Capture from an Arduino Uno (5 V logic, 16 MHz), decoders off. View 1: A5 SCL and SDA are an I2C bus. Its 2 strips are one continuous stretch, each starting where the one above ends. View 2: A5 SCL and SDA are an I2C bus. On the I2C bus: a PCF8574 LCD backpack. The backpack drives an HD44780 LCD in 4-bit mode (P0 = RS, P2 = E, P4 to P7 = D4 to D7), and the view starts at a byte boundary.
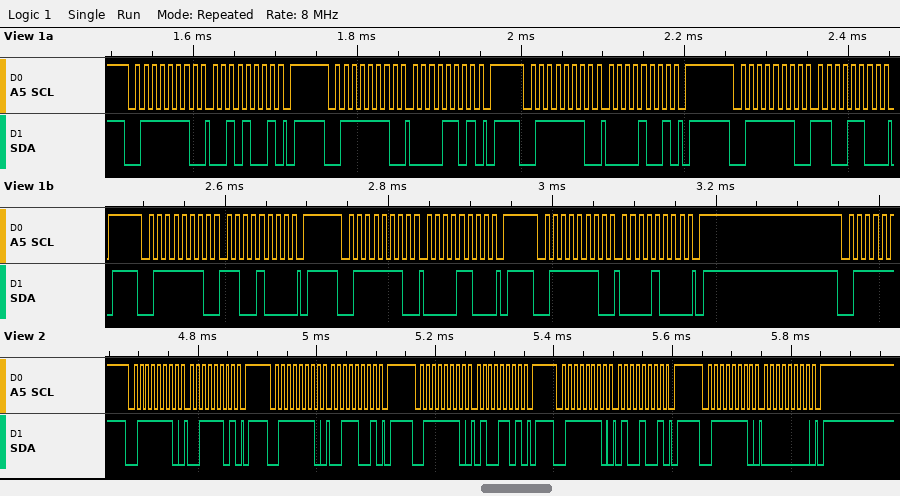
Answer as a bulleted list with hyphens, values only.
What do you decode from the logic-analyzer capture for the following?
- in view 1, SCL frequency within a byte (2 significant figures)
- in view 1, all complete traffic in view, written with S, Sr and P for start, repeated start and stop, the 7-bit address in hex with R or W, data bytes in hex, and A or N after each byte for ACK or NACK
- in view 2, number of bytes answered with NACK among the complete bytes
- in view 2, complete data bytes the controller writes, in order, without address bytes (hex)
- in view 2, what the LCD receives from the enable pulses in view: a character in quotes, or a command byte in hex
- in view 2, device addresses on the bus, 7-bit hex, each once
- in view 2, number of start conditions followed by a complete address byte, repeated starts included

- 100 kHz
- S 3FW A 29 A P S 3FW A 0D A P S 3FW A 09 A P S 3FW A CC A P S 3FW A C8 A P S 3FW A 0C A P S 3FW A 08 A P
- 0
- 3D 39 4D 49 00
- '4'
- 0x3F
- 5
